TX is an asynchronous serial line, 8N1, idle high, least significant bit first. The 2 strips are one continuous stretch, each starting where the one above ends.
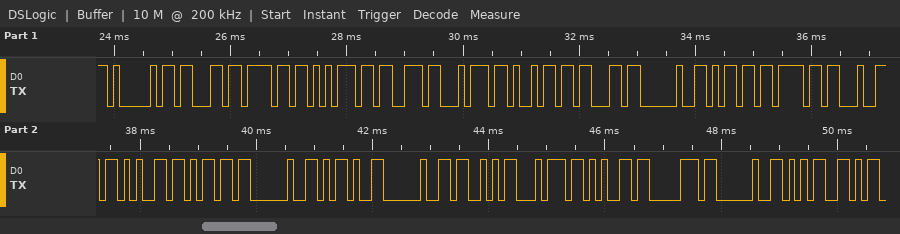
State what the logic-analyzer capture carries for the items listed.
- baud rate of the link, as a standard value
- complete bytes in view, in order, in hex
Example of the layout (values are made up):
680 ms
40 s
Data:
9600 baud
0x41 0x63 0x6F 0x75 0x73 0x74 0x69 0x63 0x20 0x6D 0x6F 0x64 0x65 0x6D 0x20 0x2D 0x20 0x53 0x74 0x65 0x70 0x20 0x35
